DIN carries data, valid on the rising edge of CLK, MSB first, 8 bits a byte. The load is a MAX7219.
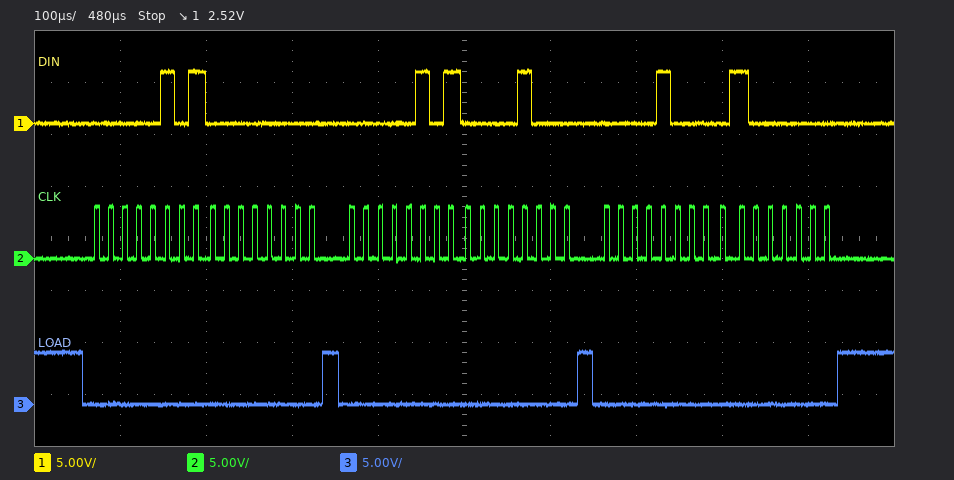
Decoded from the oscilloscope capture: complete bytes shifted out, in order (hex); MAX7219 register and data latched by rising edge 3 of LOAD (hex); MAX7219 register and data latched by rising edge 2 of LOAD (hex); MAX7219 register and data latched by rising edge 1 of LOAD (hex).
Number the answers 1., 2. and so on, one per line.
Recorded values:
1. 05 00 05 08 08 40
2. register 0x8, data 0x40
3. register 0x5, data 0x08
4. register 0x5, data 0x00
